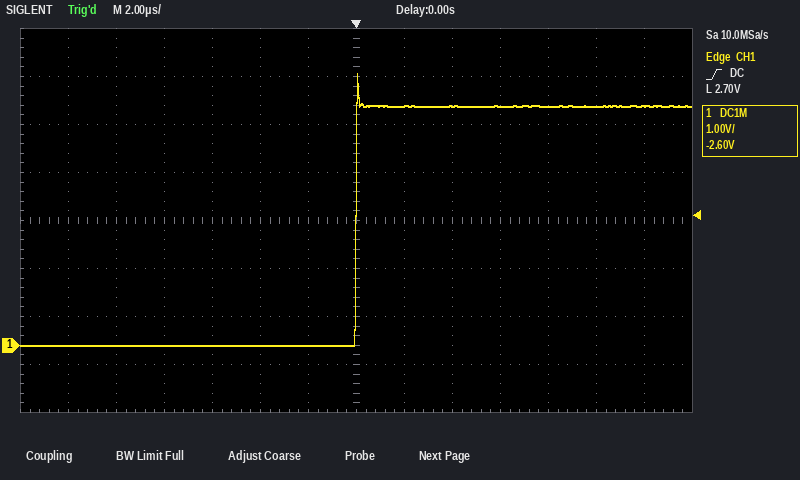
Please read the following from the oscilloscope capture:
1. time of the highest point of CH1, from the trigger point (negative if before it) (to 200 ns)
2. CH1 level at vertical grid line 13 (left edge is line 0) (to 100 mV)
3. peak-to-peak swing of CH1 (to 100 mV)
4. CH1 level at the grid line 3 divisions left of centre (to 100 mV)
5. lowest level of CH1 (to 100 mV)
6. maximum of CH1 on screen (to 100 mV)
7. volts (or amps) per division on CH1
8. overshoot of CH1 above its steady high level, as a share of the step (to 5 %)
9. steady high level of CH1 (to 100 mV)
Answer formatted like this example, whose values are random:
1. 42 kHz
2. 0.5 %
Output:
1. 0.0 µs
2. 5.0 V
3. 5.7 V
4. 0.0 V
5. 0.0 V
6. 5.7 V
7. 1 V
8. 15 %
9. 5.0 V
